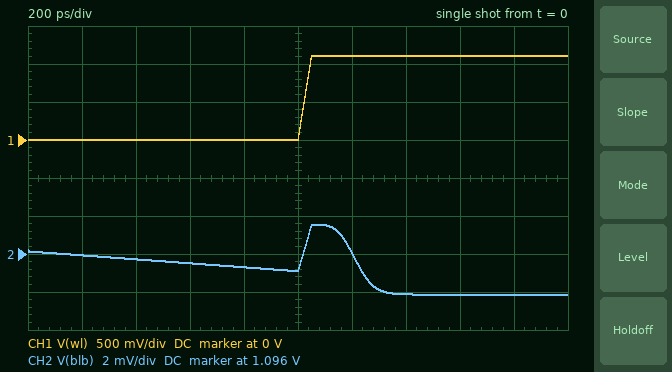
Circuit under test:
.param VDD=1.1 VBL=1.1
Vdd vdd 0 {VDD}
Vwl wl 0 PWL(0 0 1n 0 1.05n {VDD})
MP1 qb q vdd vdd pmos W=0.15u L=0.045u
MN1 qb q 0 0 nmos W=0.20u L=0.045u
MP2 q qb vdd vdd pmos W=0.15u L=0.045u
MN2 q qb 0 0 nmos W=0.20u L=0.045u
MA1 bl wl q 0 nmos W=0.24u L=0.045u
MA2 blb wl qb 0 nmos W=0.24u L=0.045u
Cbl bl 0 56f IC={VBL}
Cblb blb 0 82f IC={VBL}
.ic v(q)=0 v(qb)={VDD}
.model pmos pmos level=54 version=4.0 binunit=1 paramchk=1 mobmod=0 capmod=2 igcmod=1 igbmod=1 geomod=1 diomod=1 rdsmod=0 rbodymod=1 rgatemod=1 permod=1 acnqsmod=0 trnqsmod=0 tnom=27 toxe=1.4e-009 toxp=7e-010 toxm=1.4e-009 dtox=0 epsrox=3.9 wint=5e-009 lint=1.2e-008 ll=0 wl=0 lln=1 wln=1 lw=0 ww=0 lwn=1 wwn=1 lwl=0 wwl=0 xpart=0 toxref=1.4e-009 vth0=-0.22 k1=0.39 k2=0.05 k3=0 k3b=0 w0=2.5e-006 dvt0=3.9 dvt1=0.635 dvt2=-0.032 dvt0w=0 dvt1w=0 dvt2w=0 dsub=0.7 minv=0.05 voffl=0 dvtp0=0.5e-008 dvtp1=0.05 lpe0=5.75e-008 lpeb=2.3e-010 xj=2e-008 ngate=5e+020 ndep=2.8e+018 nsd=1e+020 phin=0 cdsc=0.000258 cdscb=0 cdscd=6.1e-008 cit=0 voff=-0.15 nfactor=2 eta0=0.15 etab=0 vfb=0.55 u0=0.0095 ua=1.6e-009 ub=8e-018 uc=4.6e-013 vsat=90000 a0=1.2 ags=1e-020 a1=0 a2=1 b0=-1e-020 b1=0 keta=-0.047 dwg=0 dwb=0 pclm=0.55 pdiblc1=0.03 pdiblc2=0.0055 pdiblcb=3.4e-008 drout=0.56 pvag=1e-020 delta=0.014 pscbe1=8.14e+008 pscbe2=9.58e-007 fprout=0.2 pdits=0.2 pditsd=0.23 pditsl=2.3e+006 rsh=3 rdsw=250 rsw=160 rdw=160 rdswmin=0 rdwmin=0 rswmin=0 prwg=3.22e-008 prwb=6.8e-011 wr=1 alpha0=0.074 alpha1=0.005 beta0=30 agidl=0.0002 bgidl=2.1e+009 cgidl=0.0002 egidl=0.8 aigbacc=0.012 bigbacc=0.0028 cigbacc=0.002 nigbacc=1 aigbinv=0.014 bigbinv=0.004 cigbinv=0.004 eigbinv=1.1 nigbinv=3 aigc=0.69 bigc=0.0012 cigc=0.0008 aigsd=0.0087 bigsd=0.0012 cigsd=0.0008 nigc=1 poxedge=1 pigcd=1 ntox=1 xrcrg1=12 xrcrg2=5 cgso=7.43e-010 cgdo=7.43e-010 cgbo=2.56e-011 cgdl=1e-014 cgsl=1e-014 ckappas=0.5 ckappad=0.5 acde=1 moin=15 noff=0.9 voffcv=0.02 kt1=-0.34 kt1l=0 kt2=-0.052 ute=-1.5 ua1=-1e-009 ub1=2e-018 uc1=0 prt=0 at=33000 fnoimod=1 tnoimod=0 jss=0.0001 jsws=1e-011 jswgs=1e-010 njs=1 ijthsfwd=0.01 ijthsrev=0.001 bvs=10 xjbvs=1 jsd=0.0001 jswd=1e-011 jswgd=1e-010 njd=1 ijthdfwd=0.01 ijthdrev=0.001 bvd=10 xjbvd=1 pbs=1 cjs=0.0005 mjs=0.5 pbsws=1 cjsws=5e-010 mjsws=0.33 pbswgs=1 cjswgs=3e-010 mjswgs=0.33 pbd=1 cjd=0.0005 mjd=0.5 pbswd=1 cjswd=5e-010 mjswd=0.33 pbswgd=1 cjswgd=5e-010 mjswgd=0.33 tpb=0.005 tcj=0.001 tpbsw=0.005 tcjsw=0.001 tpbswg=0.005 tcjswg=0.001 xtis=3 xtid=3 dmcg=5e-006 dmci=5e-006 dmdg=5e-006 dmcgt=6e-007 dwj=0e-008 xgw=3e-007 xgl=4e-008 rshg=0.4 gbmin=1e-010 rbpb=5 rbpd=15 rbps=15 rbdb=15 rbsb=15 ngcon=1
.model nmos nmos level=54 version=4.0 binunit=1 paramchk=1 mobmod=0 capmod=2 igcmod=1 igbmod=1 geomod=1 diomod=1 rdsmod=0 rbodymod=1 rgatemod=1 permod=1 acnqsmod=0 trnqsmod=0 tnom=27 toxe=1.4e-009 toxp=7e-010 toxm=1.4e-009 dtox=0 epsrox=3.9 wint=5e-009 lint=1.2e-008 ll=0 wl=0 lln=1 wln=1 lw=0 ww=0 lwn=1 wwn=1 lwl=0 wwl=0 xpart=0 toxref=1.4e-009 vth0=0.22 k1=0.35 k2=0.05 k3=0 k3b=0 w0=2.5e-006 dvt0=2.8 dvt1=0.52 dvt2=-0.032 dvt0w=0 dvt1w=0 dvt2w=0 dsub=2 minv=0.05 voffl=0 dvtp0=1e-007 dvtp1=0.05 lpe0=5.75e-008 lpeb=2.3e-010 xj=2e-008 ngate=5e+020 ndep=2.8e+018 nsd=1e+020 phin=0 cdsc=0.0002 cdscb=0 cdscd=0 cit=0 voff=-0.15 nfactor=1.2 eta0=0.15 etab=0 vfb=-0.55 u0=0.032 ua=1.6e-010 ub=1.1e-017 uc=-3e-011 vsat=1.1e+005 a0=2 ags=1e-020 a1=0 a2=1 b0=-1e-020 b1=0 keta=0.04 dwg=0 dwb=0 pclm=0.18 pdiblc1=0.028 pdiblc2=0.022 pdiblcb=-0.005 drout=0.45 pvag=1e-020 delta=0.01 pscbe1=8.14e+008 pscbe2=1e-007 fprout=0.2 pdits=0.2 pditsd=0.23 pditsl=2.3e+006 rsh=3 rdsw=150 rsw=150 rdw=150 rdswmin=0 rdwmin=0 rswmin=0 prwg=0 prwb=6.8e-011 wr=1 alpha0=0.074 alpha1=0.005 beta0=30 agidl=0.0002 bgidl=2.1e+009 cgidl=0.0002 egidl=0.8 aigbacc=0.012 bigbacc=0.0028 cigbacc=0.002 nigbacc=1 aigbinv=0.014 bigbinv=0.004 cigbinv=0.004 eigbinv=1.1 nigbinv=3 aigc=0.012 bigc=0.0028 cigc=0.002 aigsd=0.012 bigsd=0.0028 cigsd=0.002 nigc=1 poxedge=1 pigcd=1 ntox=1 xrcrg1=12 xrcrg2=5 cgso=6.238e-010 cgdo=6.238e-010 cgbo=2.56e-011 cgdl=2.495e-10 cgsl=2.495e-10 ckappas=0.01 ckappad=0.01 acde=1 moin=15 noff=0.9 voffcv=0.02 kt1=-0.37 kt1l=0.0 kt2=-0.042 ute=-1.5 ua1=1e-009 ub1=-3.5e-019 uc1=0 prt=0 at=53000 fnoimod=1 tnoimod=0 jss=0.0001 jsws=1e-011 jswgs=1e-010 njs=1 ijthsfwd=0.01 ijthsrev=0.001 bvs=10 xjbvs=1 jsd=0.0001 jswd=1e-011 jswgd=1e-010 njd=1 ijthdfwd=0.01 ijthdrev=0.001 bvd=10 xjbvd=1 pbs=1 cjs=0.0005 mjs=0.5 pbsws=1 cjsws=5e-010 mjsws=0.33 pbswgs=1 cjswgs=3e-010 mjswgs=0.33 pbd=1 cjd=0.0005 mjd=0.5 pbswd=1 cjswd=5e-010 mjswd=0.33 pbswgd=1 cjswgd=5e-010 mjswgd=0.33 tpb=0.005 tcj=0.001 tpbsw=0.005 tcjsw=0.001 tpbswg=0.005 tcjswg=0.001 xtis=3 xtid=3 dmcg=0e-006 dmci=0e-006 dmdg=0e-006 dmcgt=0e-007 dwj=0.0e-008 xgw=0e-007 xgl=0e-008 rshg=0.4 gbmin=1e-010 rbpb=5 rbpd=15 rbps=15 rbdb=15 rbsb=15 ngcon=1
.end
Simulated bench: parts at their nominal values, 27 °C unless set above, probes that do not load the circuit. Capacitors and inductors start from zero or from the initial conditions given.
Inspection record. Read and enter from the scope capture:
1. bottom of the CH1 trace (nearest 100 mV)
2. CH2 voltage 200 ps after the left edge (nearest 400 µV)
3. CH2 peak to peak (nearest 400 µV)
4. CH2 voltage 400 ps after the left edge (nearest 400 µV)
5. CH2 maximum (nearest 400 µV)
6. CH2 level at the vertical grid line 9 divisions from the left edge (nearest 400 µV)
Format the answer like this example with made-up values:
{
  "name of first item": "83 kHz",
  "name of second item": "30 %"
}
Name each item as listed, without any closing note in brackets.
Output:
{
  "bottom of the CH1 trace": "0 V",
  "CH2 voltage 200 ps after the left edge": "1.0960 V",
  "CH2 peak to peak": "3.6 mV",
  "CH2 voltage 400 ps after the left edge": "1.0956 V",
  "CH2 maximum": "1.0976 V",
  "CH2 level at the vertical grid line 9 divisions from the left edge": "1.0940 V"
}
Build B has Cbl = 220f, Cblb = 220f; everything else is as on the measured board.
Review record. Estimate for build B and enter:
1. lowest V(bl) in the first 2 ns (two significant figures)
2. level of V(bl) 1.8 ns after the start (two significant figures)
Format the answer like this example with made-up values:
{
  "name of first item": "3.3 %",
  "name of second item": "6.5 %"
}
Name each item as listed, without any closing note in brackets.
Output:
{
  "lowest V(bl) in the first 2 ns": "660 mV",
  "level of V(bl) 1.8 ns after the start": "750 mV"
}
